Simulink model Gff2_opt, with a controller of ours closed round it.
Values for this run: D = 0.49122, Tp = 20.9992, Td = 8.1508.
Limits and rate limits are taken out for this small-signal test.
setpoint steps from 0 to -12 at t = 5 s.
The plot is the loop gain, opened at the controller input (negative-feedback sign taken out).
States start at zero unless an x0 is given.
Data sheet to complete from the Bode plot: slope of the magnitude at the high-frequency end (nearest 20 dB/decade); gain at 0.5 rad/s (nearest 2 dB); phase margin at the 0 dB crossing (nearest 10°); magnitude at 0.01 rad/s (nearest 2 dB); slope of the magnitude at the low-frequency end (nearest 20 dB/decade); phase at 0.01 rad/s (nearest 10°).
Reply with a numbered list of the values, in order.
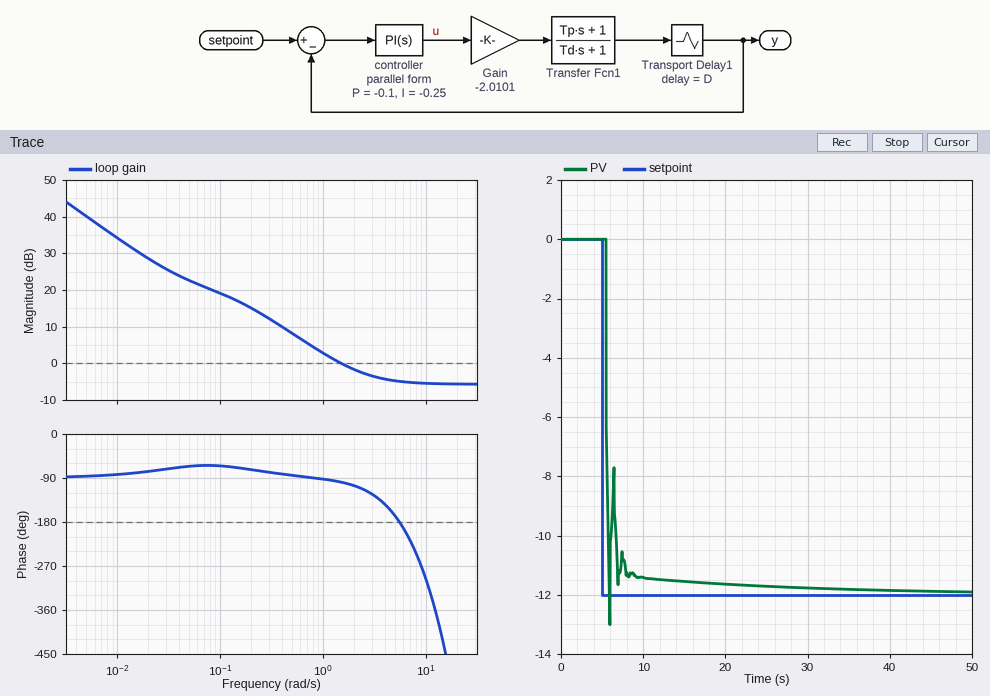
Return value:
1. 0 dB/decade
2. 8 dB
3. 80°
4. 34 dB
5. -20 dB/decade
6. -80°
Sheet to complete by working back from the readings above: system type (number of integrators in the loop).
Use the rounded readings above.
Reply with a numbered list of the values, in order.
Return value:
1. 1
